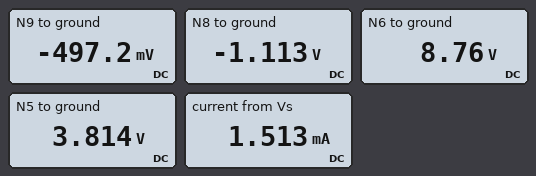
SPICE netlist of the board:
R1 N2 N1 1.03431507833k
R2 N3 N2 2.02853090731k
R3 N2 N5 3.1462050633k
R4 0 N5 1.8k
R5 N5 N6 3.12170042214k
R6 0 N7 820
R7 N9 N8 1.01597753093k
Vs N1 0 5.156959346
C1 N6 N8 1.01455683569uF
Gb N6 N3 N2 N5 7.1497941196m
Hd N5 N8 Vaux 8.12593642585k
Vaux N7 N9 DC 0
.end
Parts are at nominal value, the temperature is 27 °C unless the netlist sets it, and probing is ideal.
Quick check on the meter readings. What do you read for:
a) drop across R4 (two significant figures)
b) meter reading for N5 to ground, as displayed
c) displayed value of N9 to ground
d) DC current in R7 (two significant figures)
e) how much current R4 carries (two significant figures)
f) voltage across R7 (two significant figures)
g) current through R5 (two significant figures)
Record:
3.8 V
3.814 V
-497.2 mV
610 µA
2.1 mA
620 mV
1.6 mA
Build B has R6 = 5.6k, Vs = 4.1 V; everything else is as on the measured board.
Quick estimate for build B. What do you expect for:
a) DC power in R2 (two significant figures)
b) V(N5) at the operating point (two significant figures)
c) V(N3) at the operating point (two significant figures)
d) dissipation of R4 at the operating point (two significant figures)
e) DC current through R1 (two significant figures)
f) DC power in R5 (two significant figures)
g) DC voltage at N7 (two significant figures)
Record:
520 µW
4.5 V
5.6 V
11 mW
480 µA
800 µW
-17 V
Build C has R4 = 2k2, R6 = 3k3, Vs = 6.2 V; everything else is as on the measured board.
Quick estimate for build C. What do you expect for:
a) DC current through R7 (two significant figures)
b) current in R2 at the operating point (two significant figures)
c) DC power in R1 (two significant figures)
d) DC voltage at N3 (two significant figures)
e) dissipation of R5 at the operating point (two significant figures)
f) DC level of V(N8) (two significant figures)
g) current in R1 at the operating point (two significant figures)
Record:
1.4 mA
1.1 mA
1.1 mW
3.0 V
3.5 mW
-6.0 V
1.0 mA
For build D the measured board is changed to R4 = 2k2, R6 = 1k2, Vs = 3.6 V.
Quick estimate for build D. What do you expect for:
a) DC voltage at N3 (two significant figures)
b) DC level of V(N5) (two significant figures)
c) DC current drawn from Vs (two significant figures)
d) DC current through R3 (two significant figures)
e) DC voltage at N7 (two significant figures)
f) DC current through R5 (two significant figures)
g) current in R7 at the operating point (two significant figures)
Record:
1.0 V
2.9 V
820 µA
38 µA
-580 mV
860 µA
490 µA
